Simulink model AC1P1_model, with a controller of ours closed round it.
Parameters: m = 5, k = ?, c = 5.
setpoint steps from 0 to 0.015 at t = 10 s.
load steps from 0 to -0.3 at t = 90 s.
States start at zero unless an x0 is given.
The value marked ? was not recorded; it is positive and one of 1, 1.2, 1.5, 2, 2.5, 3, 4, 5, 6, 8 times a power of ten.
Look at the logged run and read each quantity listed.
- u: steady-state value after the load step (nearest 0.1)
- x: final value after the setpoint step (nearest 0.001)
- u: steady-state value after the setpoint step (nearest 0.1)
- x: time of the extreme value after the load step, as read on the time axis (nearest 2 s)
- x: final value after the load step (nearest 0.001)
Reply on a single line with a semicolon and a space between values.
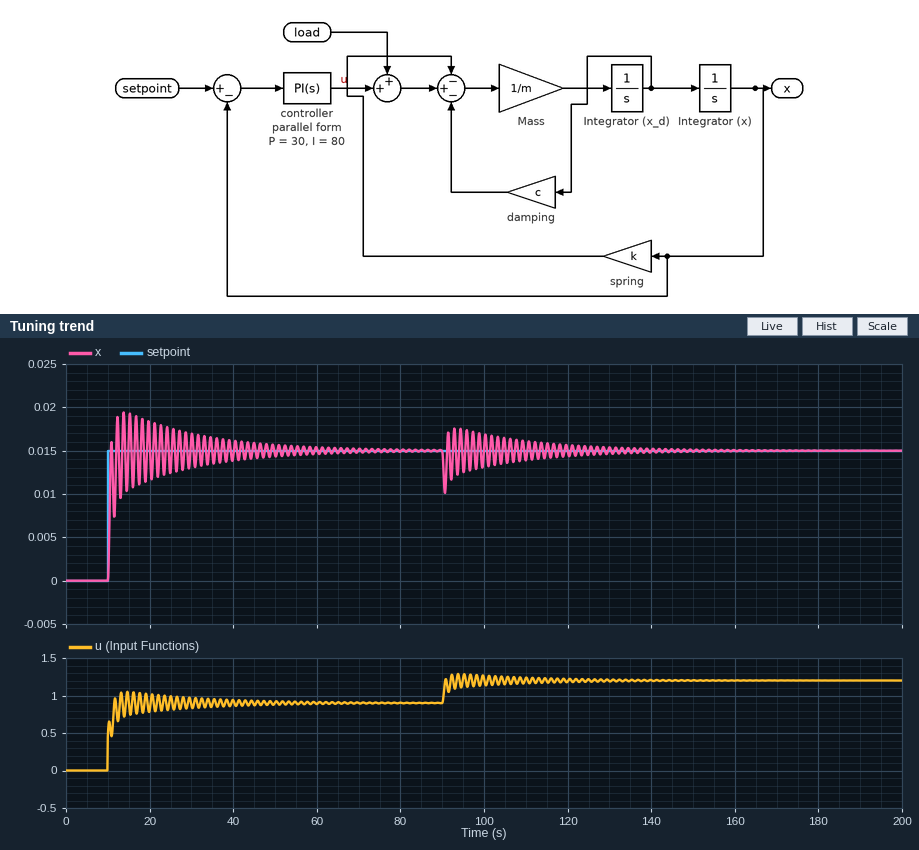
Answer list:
1.2; 0.015; 0.9; 90 s; 0.015
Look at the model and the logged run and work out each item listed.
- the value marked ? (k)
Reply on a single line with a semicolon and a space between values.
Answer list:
60
